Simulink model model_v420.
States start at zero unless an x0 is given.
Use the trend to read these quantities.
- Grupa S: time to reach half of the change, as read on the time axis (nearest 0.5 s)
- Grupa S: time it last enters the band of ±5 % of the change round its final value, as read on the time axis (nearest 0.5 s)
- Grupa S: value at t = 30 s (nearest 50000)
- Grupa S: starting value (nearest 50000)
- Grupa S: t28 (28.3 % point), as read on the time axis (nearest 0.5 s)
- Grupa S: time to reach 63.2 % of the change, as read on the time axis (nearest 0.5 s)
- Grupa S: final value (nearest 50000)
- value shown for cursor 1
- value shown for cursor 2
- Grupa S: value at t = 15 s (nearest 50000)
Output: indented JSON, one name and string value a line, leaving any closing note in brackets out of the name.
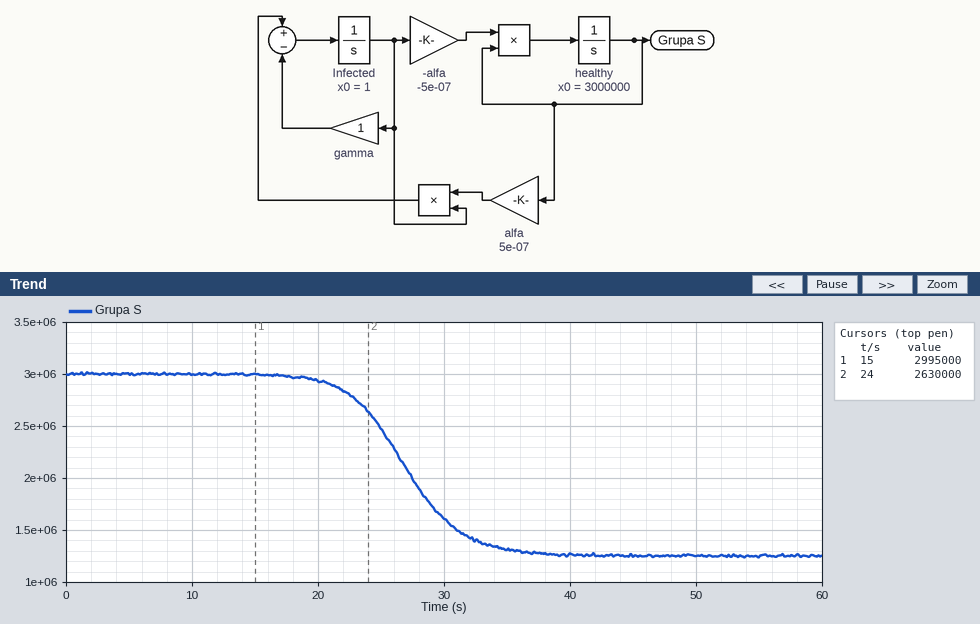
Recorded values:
{
  "Grupa S: time to reach half of the change, as read on the time axis": "27.0 s",
  "Grupa S: time it last enters the band of ±5 % of the change round its final value, as read on the time axis": "34.0 s",
  "Grupa S: value at t = 30 s": "1600000",
  "Grupa S: starting value": "3000000",
  "Grupa S: t28 (28.3 % point), as read on the time axis": "25.0 s",
  "Grupa S: time to reach 63.2 % of the change, as read on the time axis": "28.0 s",
  "Grupa S: final value": "1250000",
  "value shown for cursor 1": "2995000",
  "value shown for cursor 2": "2630000",
  "Grupa S: value at t = 15 s": "3000000"
}
